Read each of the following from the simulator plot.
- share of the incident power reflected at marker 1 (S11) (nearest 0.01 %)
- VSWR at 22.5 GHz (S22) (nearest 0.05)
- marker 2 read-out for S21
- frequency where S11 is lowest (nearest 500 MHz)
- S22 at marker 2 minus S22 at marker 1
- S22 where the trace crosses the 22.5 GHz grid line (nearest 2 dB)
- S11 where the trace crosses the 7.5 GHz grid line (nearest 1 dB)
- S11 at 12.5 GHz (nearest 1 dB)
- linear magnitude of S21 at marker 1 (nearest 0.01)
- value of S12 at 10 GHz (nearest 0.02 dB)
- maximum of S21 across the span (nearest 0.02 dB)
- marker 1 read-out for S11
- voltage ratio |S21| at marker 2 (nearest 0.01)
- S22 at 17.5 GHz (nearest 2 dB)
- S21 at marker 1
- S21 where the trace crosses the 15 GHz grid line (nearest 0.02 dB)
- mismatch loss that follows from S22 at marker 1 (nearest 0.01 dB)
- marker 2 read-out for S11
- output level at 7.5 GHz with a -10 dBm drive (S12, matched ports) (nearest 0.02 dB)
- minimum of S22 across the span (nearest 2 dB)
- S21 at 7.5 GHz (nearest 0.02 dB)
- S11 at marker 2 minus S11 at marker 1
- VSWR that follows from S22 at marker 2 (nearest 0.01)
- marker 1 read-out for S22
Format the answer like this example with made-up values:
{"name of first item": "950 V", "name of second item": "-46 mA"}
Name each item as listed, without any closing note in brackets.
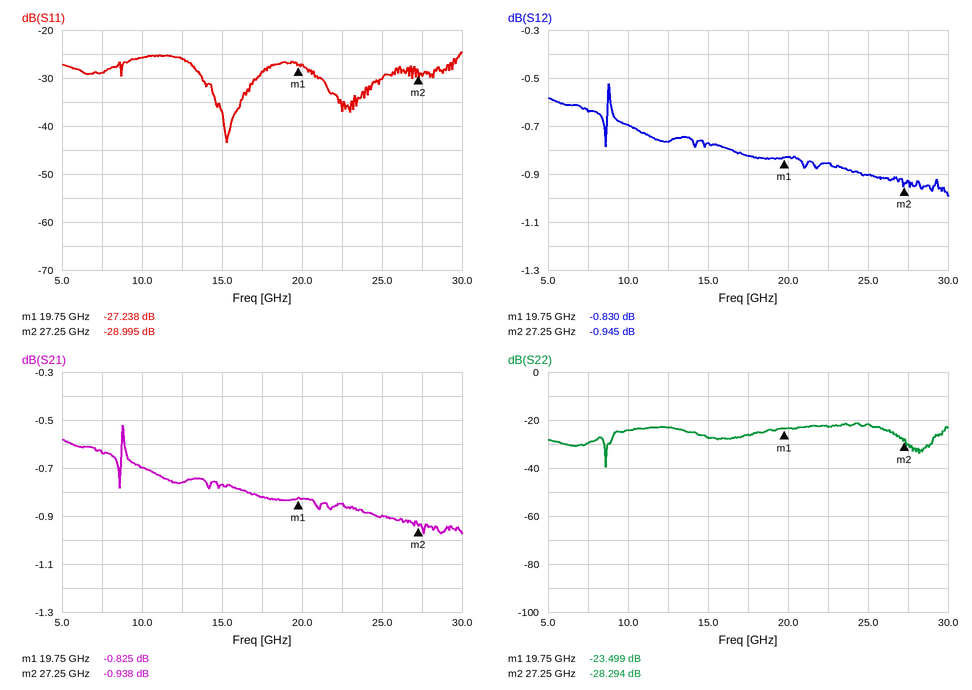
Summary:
{"share of the incident power reflected at marker 1 (S11)": "0.19 %", "VSWR at 22.5 GHz (S22)": "1.15", "marker 2 read-out for S21": "-0.938 dB", "frequency where S11 is lowest": "15.5 GHz", "S22 at marker 2 minus S22 at marker 1": "-4.795 dB", "S22 where the trace crosses the 22.5 GHz grid line": "-22 dB", "S11 where the trace crosses the 7.5 GHz grid line": "-29 dB", "S11 at 12.5 GHz": "-26 dB", "linear magnitude of S21 at marker 1": "0.91", "value of S12 at 10 GHz": "-0.70 dB", "maximum of S21 across the span": "-0.52 dB", "marker 1 read-out for S11": "-27.238 dB", "voltage ratio |S21| at marker 2": "0.90", "S22 at 17.5 GHz": "-26 dB", "S21 at marker 1": "-0.825 dB", "S21 where the trace crosses the 15 GHz grid line": "-0.76 dB", "mismatch loss that follows from S22 at marker 1": "0.02 dB", "marker 2 read-out for S11": "-28.995 dB", "output level at 7.5 GHz with a -10 dBm drive (S12, matched ports)": "-10.64 dBm", "minimum of S22 across the span": "-40 dB", "S21 at 7.5 GHz": "-0.64 dB", "S11 at marker 2 minus S11 at marker 1": "-1.757 dB", "VSWR that follows from S22 at marker 2": "1.08", "marker 1 read-out for S22": "-23.499 dB"}
